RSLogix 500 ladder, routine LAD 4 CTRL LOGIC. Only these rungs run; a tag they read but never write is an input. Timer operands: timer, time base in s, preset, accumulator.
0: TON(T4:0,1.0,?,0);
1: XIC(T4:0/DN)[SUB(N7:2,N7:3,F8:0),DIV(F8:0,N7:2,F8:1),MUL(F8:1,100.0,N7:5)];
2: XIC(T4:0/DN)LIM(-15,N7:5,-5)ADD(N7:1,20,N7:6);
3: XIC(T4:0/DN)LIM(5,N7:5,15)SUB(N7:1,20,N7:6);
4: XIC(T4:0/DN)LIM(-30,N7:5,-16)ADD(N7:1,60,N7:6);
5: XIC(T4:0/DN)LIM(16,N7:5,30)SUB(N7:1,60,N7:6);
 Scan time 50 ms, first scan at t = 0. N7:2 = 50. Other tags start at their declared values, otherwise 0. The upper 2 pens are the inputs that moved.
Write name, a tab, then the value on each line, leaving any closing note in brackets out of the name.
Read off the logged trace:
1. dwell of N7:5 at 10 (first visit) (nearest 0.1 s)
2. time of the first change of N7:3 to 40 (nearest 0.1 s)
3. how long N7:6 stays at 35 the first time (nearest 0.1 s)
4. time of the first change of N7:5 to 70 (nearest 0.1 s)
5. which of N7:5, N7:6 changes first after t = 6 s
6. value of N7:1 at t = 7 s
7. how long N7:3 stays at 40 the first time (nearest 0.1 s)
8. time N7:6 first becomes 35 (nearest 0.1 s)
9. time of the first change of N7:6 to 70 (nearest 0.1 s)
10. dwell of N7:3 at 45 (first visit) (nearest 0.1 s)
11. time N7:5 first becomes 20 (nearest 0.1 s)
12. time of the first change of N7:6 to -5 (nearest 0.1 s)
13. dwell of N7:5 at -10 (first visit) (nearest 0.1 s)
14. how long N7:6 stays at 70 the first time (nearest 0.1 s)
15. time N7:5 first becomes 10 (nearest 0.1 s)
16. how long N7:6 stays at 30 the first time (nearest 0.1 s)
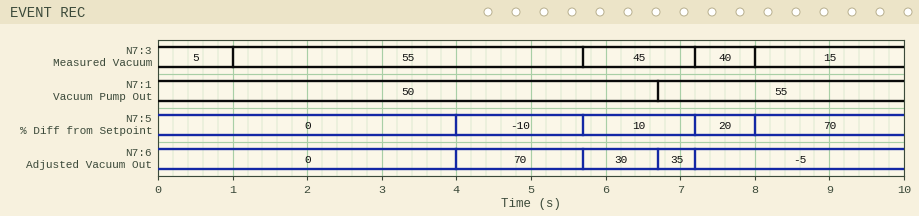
dwell of N7:5 at 10 (first visit)	1.5 s
time of the first change of N7:3 to 40	7.2 s
how long N7:6 stays at 35 the first time	0.5 s
time of the first change of N7:5 to 70	8.0 s
which of N7:5, N7:6 changes first after t = 6 s	N7:6
value of N7:1 at t = 7 s	55
how long N7:3 stays at 40 the first time	0.8 s
time N7:6 first becomes 35	6.7 s
time of the first change of N7:6 to 70	4.0 s
dwell of N7:3 at 45 (first visit)	1.5 s
time N7:5 first becomes 20	7.2 s
time of the first change of N7:6 to -5	7.2 s
dwell of N7:5 at -10 (first visit)	1.7 s
how long N7:6 stays at 70 the first time	1.7 s
time N7:5 first becomes 10	5.7 s
how long N7:6 stays at 30 the first time	1.0 s
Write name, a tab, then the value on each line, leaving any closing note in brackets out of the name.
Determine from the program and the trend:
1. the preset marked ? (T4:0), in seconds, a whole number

the preset marked ? (T4:0), in seconds, a whole number	4 s
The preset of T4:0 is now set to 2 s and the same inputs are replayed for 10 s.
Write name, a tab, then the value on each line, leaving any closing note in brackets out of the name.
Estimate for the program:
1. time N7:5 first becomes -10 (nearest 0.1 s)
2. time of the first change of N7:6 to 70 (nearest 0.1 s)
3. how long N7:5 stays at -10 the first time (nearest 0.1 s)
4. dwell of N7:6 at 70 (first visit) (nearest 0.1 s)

time N7:5 first becomes -10	2.0 s
time of the first change of N7:6 to 70	2.0 s
how long N7:5 stays at -10 the first time	3.7 s
dwell of N7:6 at 70 (first visit)	3.7 s
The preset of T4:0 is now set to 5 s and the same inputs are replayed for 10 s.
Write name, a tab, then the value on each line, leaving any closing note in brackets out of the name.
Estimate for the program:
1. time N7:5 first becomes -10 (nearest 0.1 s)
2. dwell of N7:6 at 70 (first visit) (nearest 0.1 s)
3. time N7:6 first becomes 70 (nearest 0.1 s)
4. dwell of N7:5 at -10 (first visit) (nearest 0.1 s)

time N7:5 first becomes -10	5.0 s
dwell of N7:6 at 70 (first visit)	0.7 s
time N7:6 first becomes 70	5.0 s
dwell of N7:5 at -10 (first visit)	0.7 s
